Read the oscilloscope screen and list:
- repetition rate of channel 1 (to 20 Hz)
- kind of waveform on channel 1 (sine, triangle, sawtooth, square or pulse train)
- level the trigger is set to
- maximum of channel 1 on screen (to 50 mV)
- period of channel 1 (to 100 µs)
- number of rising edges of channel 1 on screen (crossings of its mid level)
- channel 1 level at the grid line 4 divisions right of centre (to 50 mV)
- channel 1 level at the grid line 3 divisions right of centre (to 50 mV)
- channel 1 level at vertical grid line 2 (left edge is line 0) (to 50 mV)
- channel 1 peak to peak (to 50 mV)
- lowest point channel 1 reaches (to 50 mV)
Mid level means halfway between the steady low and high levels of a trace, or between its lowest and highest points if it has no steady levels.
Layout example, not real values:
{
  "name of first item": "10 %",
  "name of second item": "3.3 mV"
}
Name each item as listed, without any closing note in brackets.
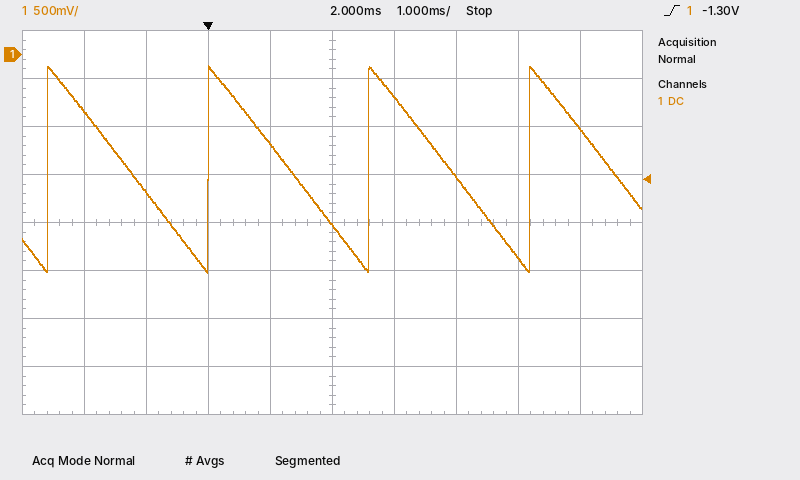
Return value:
{
  "repetition rate of channel 1": "380 Hz",
  "kind of waveform on channel 1": "sawtooth",
  "level the trigger is set to": "-1.30 V",
  "maximum of channel 1 on screen": "-100 mV",
  "period of channel 1": "2.6 ms",
  "number of rising edges of channel 1 on screen": "4",
  "channel 1 level at the grid line 4 divisions right of centre": "-750 mV",
  "channel 1 level at the grid line 3 divisions right of centre": "-2.10 V",
  "channel 1 level at vertical grid line 2 (left edge is line 0)": "-1.45 V",
  "channel 1 peak to peak": "2.15 V",
  "lowest point channel 1 reaches": "-2.25 V"
}
